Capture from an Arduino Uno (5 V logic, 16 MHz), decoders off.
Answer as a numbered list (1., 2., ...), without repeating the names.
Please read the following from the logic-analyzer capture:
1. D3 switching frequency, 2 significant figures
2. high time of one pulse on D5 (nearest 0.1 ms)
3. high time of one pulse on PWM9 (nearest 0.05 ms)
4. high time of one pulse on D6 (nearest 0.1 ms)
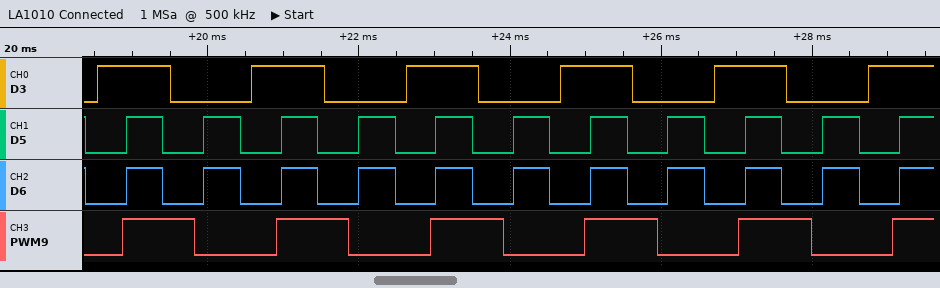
1. 490 Hz
2. 0.5 ms
3. 0.95 ms
4. 0.5 ms
